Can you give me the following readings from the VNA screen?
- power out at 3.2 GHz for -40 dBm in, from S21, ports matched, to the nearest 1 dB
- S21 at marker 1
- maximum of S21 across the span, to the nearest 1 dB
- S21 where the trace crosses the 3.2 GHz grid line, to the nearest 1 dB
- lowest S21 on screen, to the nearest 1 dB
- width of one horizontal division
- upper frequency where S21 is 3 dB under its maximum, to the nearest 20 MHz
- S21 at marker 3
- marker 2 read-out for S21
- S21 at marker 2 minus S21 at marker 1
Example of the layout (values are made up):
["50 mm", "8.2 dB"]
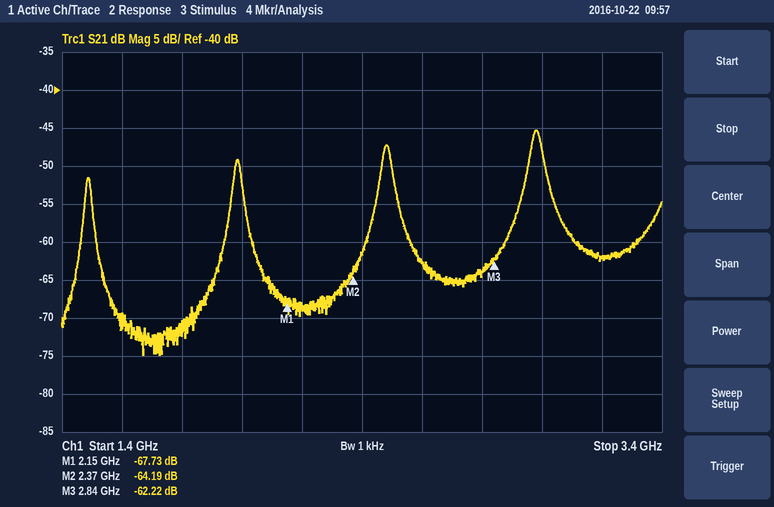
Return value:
["-102 dBm", "-67.73 dB", "-45 dB", "-62 dB", "-75 dB", "200 MHz", "3.00 GHz", "-62.22 dB", "-64.19 dB", "3.54 dB"]
